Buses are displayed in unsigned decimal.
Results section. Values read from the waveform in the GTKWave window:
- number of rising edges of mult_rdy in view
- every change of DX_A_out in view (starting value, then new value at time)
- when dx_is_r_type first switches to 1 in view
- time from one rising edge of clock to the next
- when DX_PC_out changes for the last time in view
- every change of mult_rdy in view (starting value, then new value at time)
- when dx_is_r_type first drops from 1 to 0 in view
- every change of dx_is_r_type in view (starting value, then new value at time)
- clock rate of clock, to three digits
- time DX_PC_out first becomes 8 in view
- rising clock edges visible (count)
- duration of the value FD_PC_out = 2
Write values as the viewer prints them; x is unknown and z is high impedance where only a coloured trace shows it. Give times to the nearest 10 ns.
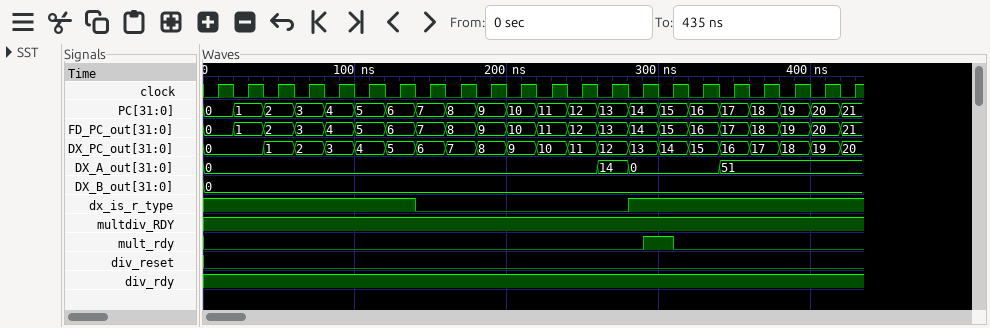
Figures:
1
0, 14 at 260 ns, 0 at 280 ns, 51 at 340 ns
280 ns
20 ns
420 ns
0, 1 at 290 ns, 0 at 310 ns
140 ns
1, 0 at 140 ns, 1 at 280 ns
50.0 MHz
180 ns
22
20 ns
